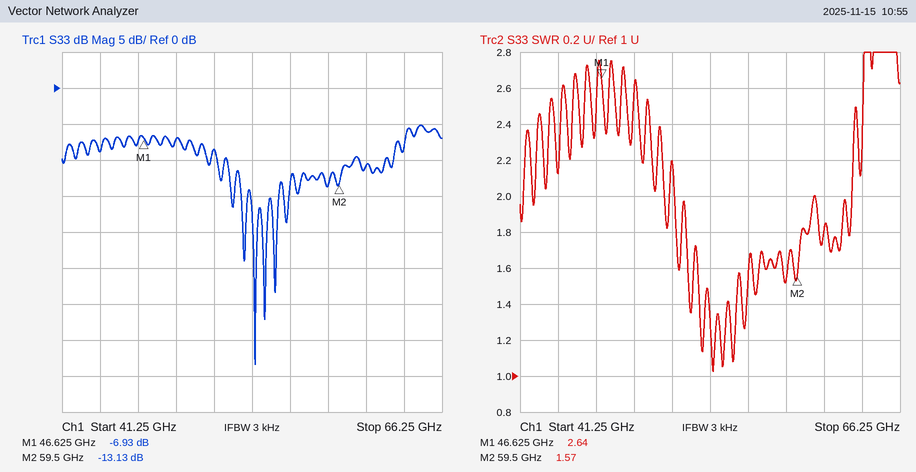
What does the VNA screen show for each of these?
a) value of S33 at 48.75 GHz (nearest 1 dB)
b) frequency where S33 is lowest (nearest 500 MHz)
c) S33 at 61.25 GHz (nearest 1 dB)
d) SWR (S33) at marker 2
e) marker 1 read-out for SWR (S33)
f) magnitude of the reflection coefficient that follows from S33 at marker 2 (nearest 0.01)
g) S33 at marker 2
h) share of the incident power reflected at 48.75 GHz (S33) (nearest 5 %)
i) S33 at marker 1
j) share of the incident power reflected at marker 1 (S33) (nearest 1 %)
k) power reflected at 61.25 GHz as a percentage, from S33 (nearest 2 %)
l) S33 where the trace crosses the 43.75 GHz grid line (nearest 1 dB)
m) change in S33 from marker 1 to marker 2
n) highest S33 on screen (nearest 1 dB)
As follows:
-7 dB
54.0 GHz
-11 dB
1.57
2.64
0.22
-13.13 dB
20 %
-6.93 dB
20 %
8 %
-9 dB
-6.20 dB
-5 dB
